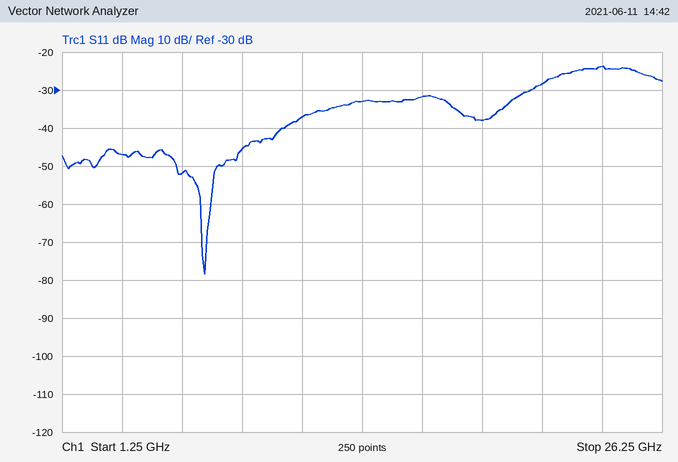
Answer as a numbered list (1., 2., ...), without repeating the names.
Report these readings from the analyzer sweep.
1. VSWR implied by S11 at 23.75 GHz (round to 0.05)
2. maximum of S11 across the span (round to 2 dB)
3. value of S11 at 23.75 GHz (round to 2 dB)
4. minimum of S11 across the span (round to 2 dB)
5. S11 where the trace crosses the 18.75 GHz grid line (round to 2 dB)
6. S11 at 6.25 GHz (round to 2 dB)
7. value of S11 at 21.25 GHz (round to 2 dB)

1. 1.15
2. -24 dB
3. -24 dB
4. -78 dB
5. -38 dB
6. -52 dB
7. -28 dB
